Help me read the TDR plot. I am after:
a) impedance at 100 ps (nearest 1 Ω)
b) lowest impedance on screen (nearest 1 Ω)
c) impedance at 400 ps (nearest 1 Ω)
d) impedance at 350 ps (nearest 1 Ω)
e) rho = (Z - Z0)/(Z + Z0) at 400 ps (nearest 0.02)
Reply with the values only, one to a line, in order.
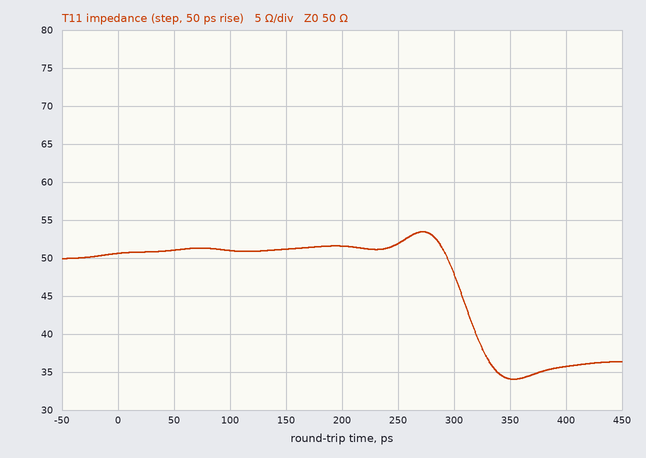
51 Ω
34 Ω
36 Ω
34 Ω
-0.16
